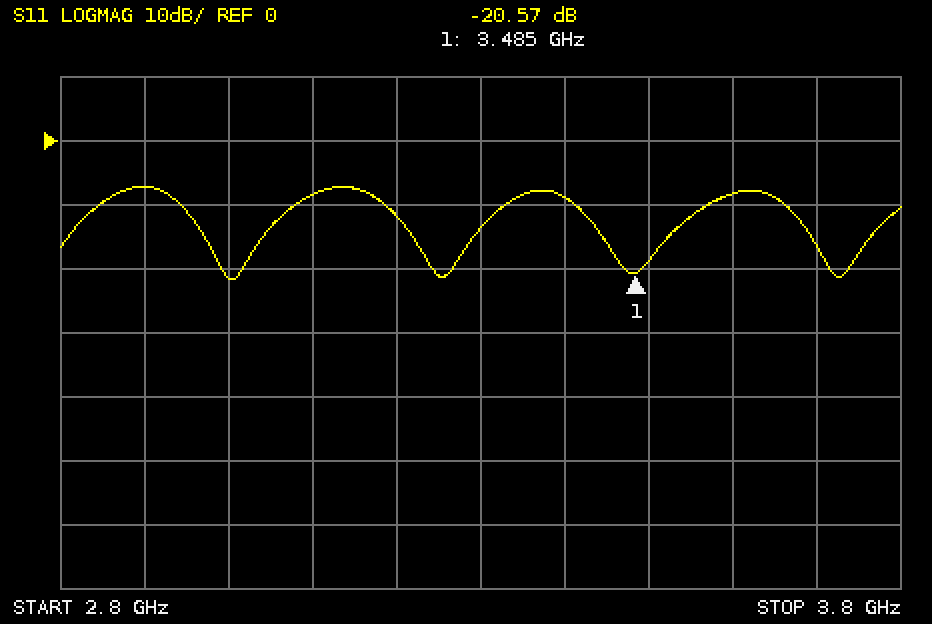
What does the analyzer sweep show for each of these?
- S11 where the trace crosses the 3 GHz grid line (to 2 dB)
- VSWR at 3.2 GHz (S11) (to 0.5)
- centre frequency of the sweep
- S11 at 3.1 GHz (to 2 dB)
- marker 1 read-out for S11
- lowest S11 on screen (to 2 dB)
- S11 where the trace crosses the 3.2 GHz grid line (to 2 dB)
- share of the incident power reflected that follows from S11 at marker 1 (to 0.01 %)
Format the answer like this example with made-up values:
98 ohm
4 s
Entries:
-22 dB
1.5
3.3 GHz
-8 dB
-20.57 dB
-22 dB
-12 dB
0.88 %
